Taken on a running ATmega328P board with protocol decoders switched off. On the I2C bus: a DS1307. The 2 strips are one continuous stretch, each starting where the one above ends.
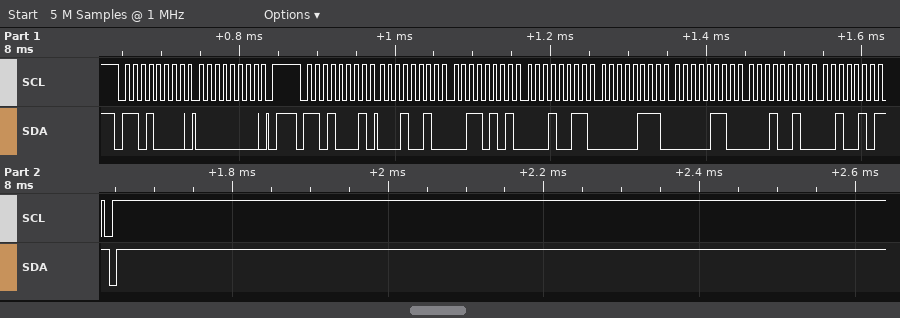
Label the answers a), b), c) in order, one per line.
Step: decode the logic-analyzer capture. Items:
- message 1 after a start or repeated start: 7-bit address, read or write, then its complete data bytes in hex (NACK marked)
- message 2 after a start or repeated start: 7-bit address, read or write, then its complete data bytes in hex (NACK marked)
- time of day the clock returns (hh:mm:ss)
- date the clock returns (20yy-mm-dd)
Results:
a) 0x68 write: 00
b) 0x68 read: 12 35 13 07 06 12 25 NACK
c) 13:35:12
d) 2025-12-06
